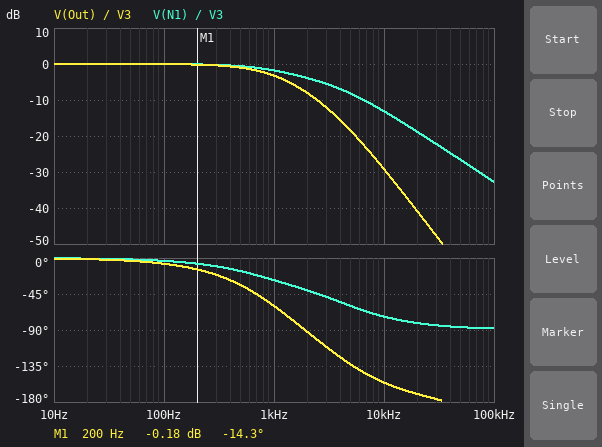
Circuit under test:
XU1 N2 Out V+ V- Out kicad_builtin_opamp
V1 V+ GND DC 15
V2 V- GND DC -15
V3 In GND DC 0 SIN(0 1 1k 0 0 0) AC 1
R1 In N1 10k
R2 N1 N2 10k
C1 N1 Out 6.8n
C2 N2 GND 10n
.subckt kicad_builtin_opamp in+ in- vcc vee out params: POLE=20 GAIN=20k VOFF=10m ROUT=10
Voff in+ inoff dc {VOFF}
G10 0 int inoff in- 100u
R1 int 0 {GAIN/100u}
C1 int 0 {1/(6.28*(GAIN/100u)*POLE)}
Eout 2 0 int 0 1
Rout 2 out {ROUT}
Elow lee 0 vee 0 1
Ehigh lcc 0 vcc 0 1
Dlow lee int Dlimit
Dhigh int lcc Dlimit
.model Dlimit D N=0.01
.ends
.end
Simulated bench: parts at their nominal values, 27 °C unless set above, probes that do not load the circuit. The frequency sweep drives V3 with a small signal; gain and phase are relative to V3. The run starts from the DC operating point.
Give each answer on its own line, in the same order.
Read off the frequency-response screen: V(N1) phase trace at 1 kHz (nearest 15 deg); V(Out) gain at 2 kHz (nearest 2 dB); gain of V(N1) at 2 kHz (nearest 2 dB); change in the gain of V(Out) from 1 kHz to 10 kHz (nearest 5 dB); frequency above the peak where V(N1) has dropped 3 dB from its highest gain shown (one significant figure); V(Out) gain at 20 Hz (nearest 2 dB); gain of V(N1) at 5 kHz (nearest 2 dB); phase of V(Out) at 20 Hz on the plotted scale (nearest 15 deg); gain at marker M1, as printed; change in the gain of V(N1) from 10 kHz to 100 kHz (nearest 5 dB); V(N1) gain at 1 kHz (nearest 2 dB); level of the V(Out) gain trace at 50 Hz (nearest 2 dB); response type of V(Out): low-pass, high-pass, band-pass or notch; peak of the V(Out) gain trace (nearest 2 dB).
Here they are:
-30 deg
-8 dB
-4 dB
-25 dB
2 kHz
0 dB
-8 dB
0 deg
-0.18 dB
-20 dB
-2 dB
0 dB
low-pass
0 dB
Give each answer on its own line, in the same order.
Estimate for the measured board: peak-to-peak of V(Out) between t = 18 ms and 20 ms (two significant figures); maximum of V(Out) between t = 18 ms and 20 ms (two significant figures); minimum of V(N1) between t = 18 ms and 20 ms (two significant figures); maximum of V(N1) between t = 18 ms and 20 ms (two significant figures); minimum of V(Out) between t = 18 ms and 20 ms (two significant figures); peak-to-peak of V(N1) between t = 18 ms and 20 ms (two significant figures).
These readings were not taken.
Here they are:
1.4 V
680 mV
-810 mV
810 mV
-700 mV
1.6 V
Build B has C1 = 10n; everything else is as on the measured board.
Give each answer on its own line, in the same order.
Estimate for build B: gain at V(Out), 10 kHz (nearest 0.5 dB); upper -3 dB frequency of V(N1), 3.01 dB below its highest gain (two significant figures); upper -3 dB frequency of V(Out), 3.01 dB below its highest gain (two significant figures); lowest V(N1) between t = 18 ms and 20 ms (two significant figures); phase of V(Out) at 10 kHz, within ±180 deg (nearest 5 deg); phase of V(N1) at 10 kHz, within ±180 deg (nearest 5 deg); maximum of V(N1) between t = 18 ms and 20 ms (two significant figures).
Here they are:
-32.0 dB
1.6 kHz
1.0 kHz
-850 mV
-165 deg
-80 deg
850 mV
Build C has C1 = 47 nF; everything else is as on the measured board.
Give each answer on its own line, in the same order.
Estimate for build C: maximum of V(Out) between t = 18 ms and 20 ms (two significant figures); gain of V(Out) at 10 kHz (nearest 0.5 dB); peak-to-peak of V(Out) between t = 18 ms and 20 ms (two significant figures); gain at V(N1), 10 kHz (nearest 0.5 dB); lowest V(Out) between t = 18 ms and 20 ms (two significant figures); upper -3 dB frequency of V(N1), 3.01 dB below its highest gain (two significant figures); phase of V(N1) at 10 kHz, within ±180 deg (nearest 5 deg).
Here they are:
650 mV
-45.5 dB
1.3 V
-29.5 dB
-670 mV
900 Hz
-95 deg
